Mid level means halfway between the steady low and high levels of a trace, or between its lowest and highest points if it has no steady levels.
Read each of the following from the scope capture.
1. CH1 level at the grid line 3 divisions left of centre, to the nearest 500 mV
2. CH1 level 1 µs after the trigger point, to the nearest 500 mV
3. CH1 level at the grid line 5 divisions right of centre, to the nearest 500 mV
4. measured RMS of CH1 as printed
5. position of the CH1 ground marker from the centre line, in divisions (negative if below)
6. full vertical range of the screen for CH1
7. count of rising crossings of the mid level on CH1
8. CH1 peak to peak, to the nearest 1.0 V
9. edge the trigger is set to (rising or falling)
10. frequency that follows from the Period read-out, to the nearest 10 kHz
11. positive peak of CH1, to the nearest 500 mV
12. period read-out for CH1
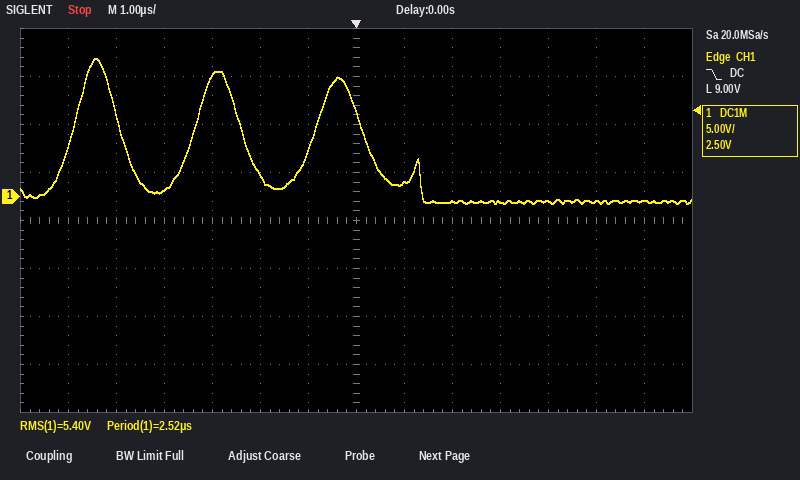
12.5 V
1.5 V
-500 mV
5.40 V
+0.5 div
40 V
3
15.0 V
falling
400 kHz
14.5 V
2.52 µs
